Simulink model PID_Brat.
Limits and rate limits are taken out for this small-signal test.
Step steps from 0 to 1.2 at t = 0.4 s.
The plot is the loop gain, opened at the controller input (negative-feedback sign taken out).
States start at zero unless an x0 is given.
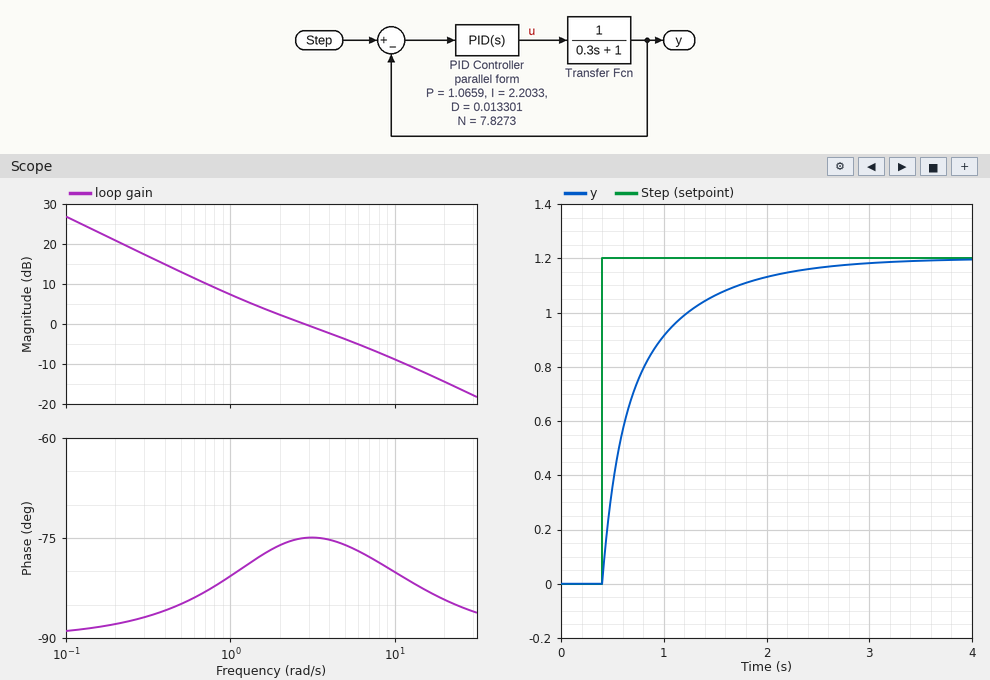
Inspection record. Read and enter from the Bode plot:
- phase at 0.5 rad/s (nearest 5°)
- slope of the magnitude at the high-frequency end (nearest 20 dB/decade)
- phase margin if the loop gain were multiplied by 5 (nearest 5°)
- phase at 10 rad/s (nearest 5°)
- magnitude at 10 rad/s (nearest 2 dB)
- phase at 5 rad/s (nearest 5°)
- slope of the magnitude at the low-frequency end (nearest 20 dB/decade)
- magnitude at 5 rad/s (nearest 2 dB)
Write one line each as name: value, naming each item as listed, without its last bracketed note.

phase at 0.5 rad/s: -85°
slope of the magnitude at the high-frequency end: -20 dB/decade
phase margin if the loop gain were multiplied by 5: 95°
phase at 10 rad/s: -80°
magnitude at 10 rad/s: -8 dB
phase at 5 rad/s: -75°
slope of the magnitude at the low-frequency end: -20 dB/decade
magnitude at 5 rad/s: -4 dB
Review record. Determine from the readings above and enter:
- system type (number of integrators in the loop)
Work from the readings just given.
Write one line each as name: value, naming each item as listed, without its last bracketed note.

system type: 1
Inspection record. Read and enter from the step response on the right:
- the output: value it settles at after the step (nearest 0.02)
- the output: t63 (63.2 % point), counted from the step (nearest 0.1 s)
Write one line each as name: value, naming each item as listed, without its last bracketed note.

the output: value it settles at after the step: 1.20
the output: t63 (63.2 % point), counted from the step: 0.4 s
